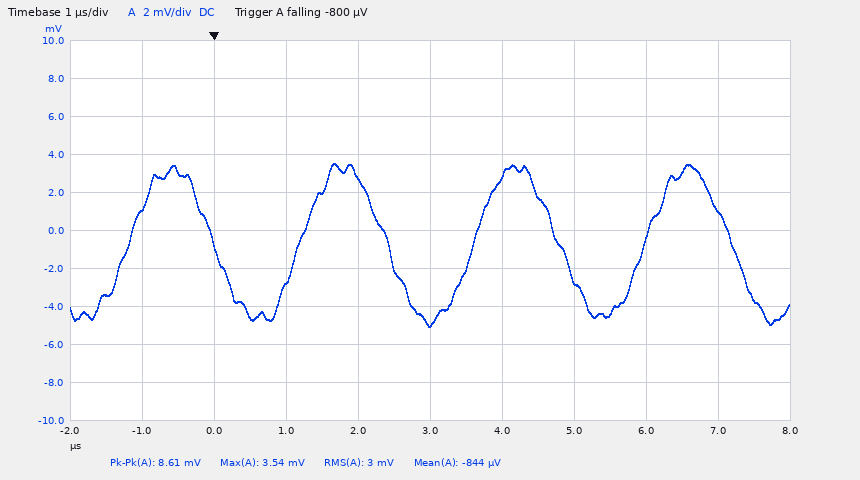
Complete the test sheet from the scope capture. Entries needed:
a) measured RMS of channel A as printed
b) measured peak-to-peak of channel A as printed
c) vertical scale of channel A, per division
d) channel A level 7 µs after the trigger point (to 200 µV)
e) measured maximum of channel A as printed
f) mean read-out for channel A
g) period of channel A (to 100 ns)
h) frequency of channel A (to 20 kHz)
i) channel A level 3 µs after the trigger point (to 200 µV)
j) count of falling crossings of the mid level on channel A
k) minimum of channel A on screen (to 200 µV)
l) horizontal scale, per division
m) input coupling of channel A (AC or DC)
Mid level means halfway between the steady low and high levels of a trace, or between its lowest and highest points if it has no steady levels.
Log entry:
3 mV
8.61 mV
2 mV
1.0 mV
3.54 mV
-844 µV
2.4 µs
420 kHz
-5.0 mV
4
-5.0 mV
1 µs
DC
